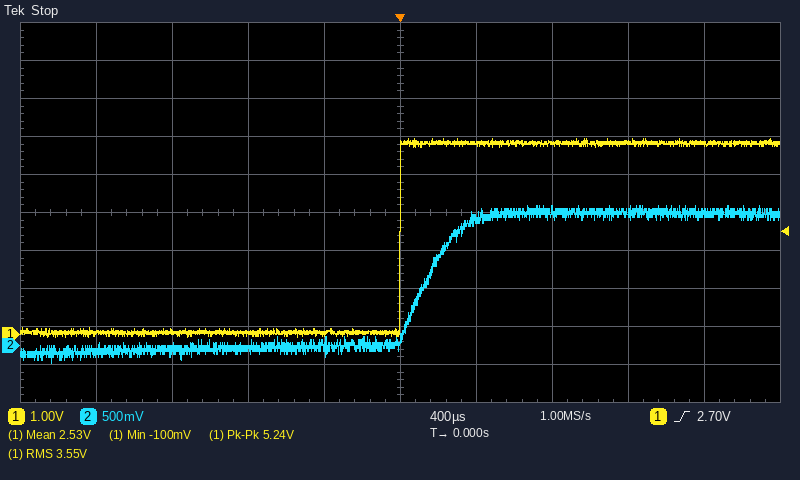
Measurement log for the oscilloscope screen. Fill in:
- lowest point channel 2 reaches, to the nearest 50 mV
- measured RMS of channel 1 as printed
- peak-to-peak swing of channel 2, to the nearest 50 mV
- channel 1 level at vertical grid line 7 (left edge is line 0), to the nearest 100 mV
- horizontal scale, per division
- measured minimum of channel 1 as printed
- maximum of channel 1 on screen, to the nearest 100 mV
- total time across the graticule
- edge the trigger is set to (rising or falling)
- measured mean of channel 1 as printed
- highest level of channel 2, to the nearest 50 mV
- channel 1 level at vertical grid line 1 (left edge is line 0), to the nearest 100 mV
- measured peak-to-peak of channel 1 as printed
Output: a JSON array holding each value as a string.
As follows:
["-250 mV", "3.55 V", "2.10 V", "5.0 V", "400 µs", "-100 mV", "5.1 V", "4 ms", "rising", "2.53 V", "1.85 V", "0.0 V", "5.24 V"]
